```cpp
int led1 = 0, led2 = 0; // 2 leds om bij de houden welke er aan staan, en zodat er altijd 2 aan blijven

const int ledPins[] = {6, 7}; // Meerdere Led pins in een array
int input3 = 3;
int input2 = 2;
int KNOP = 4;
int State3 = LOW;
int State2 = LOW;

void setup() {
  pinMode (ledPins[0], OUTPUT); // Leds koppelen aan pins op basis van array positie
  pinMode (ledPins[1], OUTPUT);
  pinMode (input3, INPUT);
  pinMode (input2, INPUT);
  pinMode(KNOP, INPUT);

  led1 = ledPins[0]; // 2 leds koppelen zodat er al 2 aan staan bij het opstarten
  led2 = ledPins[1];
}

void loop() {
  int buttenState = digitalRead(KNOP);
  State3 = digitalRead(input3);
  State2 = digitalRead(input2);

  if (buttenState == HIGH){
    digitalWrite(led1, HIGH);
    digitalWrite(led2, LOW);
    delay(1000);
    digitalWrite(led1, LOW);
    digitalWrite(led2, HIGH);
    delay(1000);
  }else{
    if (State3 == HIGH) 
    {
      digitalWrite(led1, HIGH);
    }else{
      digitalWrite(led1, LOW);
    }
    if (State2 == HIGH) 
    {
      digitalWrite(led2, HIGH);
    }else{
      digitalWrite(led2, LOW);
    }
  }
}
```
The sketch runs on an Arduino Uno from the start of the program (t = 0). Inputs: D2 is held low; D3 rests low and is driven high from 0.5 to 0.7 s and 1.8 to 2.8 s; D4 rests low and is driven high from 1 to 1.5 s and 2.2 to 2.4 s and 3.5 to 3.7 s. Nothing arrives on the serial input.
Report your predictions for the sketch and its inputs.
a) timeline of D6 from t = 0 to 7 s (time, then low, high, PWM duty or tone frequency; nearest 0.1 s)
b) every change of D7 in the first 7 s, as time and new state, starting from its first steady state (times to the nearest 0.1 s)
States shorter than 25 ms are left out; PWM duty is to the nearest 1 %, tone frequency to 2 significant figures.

0 s low; 0.5 s high; 0.7 s low; 1 s high; 2 s low; 3.5 s high; 4.5 s low
0 s low; 2 s high; 3 s low; 4.5 s high; 5.5 s low
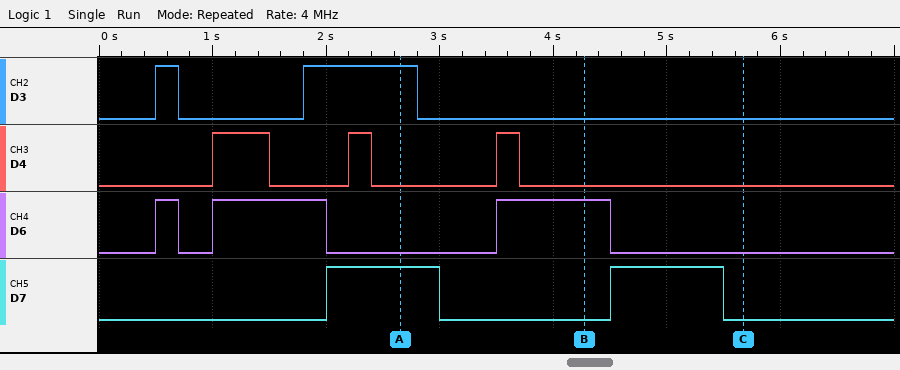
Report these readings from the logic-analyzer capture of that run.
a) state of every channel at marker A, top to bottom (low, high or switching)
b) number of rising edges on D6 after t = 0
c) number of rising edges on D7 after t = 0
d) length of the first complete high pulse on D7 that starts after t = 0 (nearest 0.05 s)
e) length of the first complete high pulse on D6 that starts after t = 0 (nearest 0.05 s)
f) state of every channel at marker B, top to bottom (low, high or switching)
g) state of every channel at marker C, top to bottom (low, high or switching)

D3 high, D4 low, D6 low, D7 high
3
2
1.00 s
0.20 s
D3 low, D4 low, D6 high, D7 low
D3 low, D4 low, D6 low, D7 low
